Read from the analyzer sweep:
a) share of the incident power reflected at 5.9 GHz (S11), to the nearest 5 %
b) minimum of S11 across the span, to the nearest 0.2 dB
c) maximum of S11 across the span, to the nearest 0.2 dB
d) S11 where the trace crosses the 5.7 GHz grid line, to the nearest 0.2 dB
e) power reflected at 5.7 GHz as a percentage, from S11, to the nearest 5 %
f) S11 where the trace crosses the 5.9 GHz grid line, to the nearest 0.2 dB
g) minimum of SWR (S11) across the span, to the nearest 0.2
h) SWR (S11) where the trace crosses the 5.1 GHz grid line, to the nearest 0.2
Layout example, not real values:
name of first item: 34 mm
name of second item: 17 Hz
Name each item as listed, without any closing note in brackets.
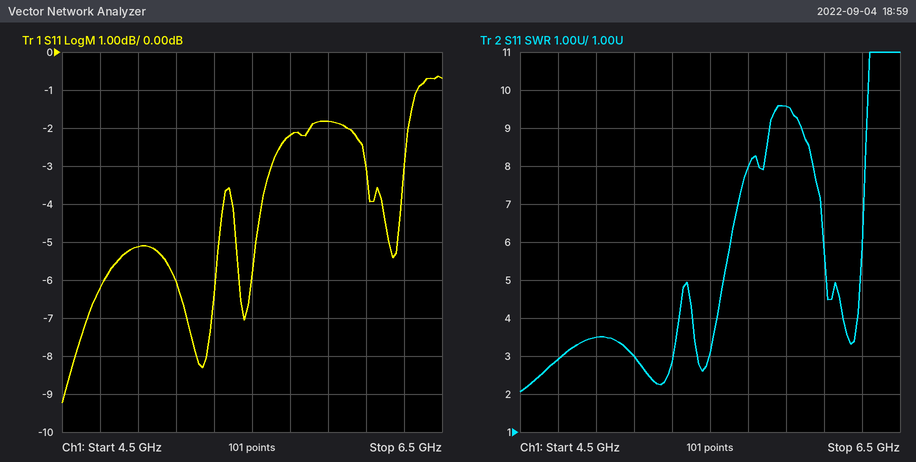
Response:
share of the incident power reflected at 5.9 GHz (S11), to the nearest 5 %: 65 %
minimum of S11 across the span, to the nearest 0.2 dB: -9.2 dB
maximum of S11 across the span, to the nearest 0.2 dB: -0.6 dB
S11 where the trace crosses the 5.7 GHz grid line, to the nearest 0.2 dB: -2.2 dB
power reflected at 5.7 GHz as a percentage, from S11, to the nearest 5 %: 60 %
S11 where the trace crosses the 5.9 GHz grid line, to the nearest 0.2 dB: -1.8 dB
minimum of SWR (S11) across the span, to the nearest 0.2: 2.0
SWR (S11) where the trace crosses the 5.1 GHz grid line, to the nearest 0.2: 3.0
